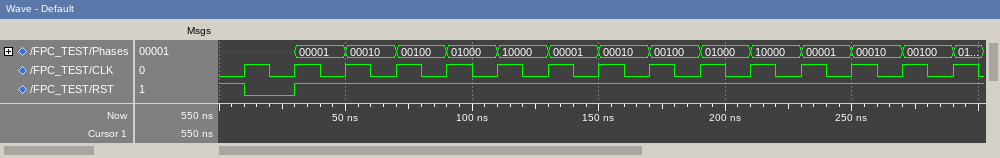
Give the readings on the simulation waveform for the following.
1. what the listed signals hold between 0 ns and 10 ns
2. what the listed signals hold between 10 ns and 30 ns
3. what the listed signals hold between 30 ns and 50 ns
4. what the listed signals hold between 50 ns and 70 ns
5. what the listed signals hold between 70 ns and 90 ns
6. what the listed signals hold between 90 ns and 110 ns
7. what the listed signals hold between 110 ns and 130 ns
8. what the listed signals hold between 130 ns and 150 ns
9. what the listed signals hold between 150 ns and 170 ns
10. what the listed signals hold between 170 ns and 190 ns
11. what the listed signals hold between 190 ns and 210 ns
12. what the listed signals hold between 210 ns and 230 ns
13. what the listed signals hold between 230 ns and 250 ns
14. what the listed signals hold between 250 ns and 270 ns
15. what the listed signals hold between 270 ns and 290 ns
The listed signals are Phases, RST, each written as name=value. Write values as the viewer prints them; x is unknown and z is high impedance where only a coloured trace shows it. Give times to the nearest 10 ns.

Phases=x, RST=1
Phases=x, RST=0
Phases=00001, RST=1
Phases=00010, RST=1
Phases=00100, RST=1
Phases=01000, RST=1
Phases=10000, RST=1
Phases=00001, RST=1
Phases=00010, RST=1
Phases=00100, RST=1
Phases=01000, RST=1
Phases=10000, RST=1
Phases=00001, RST=1
Phases=00010, RST=1
Phases=00100, RST=1
